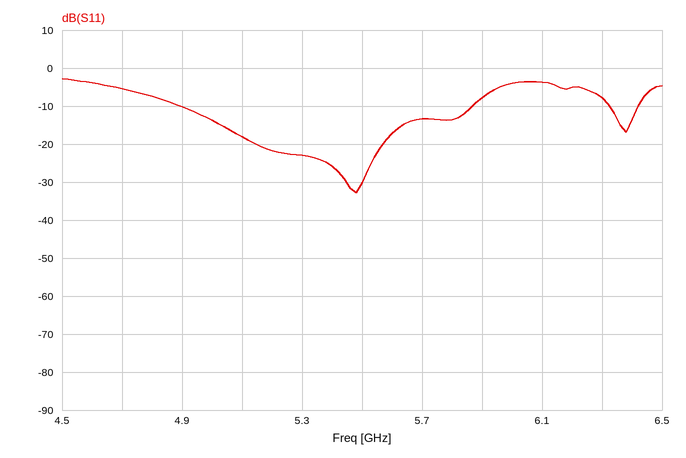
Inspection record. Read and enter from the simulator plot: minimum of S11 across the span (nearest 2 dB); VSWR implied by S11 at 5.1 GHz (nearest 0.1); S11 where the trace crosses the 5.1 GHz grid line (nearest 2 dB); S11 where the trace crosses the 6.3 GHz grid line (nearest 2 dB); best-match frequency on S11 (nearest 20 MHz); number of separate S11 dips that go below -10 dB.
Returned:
-32 dB
1.3
-18 dB
-8 dB
5.48 GHz
2
